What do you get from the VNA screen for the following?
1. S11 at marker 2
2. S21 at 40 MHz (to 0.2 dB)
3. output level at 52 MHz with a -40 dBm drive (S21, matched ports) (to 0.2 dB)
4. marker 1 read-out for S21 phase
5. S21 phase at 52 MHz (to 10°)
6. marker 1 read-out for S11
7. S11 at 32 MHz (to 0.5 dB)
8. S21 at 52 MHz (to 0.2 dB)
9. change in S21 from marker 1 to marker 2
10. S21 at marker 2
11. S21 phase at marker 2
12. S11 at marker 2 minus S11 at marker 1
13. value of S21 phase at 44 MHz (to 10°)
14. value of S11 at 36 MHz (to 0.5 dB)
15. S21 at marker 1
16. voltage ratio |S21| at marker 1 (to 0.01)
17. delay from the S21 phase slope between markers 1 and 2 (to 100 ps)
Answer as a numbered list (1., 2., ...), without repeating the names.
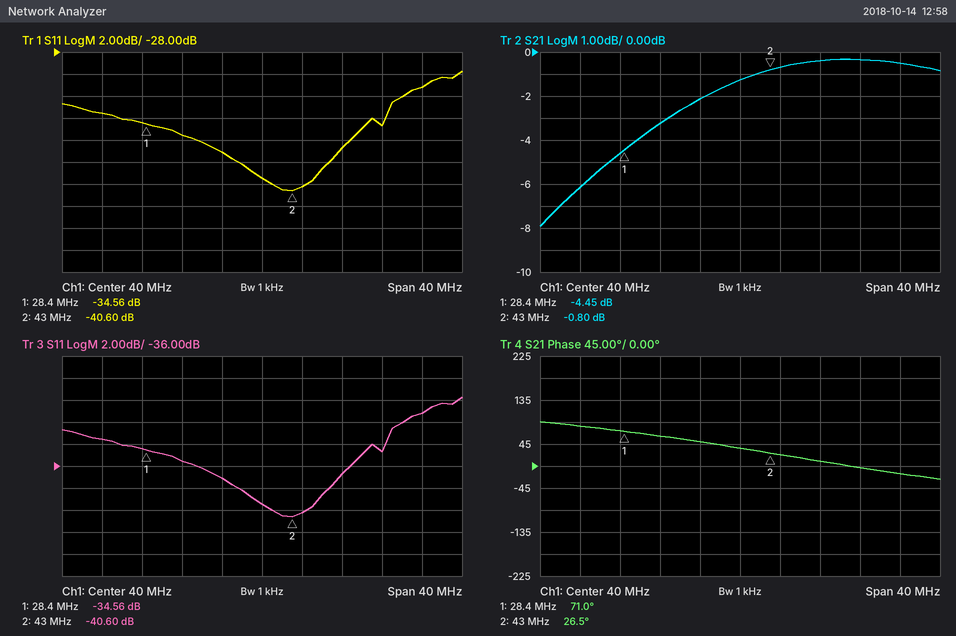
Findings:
1. -40.60 dB
2. -1.2 dB
3. -40.4 dBm
4. 71.0°
5. 0°
6. -34.56 dB
7. -35.5 dB
8. -0.4 dB
9. 3.65 dB
10. -0.80 dB
11. 26.5°
12. -6.04 dB
13. 20°
14. -37.0 dB
15. -4.45 dB
16. 0.60
17. 8.5 ns
